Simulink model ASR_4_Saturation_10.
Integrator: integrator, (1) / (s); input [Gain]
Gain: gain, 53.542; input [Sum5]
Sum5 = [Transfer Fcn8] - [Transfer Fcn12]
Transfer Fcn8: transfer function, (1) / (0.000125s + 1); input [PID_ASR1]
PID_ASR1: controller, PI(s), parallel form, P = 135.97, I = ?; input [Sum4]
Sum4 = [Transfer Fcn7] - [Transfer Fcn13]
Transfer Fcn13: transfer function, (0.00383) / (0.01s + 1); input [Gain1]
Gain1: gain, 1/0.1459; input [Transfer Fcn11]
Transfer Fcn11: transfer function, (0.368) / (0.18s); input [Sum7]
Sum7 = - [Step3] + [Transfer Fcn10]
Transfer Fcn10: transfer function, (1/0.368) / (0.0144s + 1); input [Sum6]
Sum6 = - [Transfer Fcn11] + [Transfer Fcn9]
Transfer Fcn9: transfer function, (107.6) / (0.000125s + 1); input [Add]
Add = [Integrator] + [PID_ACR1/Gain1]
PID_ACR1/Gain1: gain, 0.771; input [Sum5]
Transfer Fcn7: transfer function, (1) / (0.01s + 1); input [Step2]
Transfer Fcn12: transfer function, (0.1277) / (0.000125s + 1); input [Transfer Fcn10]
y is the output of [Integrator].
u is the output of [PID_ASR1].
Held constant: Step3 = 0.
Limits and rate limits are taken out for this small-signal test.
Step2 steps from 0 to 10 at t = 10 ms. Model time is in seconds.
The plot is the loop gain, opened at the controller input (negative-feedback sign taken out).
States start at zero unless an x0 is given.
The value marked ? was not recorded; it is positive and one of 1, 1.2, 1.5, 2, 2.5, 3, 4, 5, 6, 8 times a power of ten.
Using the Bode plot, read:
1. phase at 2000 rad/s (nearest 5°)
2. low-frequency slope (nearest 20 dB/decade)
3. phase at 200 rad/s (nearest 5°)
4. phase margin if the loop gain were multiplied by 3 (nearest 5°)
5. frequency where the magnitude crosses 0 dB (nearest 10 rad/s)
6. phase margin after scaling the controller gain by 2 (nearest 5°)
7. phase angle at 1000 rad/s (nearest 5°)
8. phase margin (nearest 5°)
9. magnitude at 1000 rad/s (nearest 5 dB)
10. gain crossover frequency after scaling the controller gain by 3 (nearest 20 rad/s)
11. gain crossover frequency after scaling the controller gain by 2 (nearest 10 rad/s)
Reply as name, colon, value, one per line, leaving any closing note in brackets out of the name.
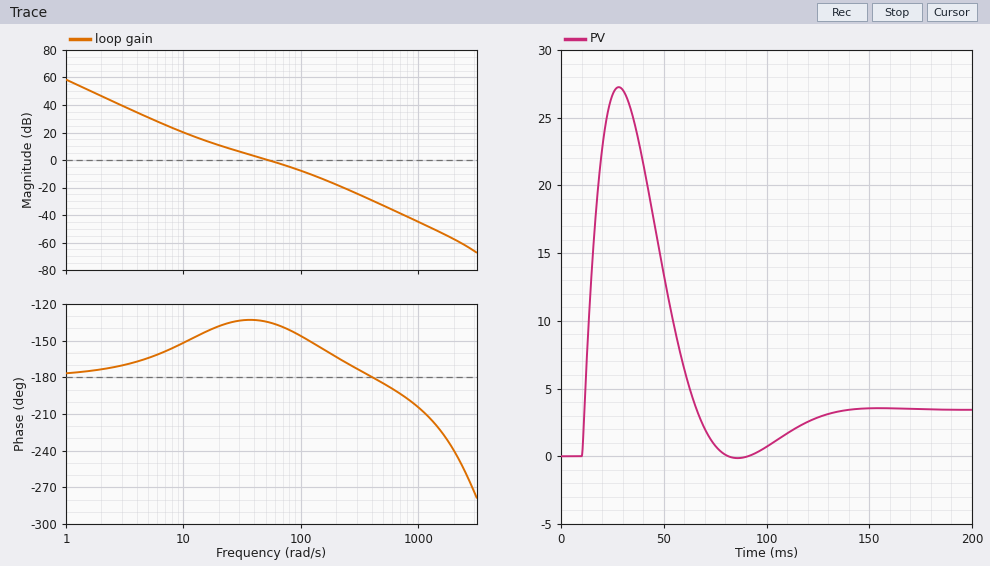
phase at 2000 rad/s: -240°
low-frequency slope: -40 dB/decade
phase at 200 rad/s: -165°
phase margin if the loop gain were multiplied by 3: 30°
frequency where the magnitude crosses 0 dB: 50 rad/s
phase margin after scaling the controller gain by 2: 35°
phase angle at 1000 rad/s: -205°
phase margin: 45°
magnitude at 1000 rad/s: -45 dB
gain crossover frequency after scaling the controller gain by 3: 120 rad/s
gain crossover frequency after scaling the controller gain by 2: 90 rad/s
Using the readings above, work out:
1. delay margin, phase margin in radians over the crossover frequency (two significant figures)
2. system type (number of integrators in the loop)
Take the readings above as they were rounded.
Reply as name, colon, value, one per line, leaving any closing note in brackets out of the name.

delay margin, phase margin in radians over the crossover frequency: 0.016 s
system type: 2
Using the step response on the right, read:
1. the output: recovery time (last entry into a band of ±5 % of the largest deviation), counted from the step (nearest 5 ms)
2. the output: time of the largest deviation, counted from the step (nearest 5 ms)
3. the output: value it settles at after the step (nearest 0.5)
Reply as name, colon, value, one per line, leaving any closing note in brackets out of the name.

the output: recovery time (last entry into a band of ±5 % of the largest deviation), counted from the step: 105 ms
the output: time of the largest deviation, counted from the step: 20 ms
the output: value it settles at after the step: 3.5
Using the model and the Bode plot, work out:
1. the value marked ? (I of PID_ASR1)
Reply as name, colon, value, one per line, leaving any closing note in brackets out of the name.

the value marked ?: 2000
